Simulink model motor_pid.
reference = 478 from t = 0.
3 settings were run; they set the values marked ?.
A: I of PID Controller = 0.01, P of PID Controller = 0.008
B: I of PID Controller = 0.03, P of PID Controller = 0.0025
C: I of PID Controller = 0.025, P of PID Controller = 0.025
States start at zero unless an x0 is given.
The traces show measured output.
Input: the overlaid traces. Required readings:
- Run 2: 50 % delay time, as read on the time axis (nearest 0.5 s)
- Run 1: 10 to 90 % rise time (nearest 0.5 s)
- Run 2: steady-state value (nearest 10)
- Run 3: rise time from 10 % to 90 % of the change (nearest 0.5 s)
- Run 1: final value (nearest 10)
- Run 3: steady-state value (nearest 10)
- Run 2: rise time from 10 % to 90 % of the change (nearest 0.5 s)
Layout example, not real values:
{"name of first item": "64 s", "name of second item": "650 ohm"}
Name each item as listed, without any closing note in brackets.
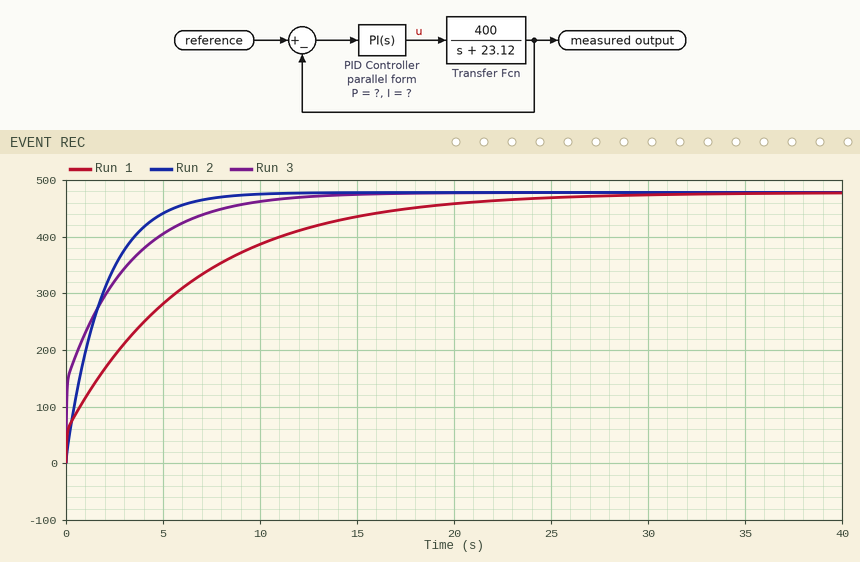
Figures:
{"Run 2: 50 % delay time, as read on the time axis": "1.5 s", "Run 1: 10 to 90 % rise time": "14.0 s", "Run 2: steady-state value": "480", "Run 3: rise time from 10 % to 90 % of the change": "6.5 s", "Run 1: final value": "480", "Run 3: steady-state value": "480", "Run 2: rise time from 10 % to 90 % of the change": "4.5 s"}
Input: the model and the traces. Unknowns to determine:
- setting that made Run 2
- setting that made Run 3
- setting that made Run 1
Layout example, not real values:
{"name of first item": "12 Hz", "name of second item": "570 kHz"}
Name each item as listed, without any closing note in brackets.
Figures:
{"setting that made Run 2": "B", "setting that made Run 3": "C", "setting that made Run 1": "A"}
